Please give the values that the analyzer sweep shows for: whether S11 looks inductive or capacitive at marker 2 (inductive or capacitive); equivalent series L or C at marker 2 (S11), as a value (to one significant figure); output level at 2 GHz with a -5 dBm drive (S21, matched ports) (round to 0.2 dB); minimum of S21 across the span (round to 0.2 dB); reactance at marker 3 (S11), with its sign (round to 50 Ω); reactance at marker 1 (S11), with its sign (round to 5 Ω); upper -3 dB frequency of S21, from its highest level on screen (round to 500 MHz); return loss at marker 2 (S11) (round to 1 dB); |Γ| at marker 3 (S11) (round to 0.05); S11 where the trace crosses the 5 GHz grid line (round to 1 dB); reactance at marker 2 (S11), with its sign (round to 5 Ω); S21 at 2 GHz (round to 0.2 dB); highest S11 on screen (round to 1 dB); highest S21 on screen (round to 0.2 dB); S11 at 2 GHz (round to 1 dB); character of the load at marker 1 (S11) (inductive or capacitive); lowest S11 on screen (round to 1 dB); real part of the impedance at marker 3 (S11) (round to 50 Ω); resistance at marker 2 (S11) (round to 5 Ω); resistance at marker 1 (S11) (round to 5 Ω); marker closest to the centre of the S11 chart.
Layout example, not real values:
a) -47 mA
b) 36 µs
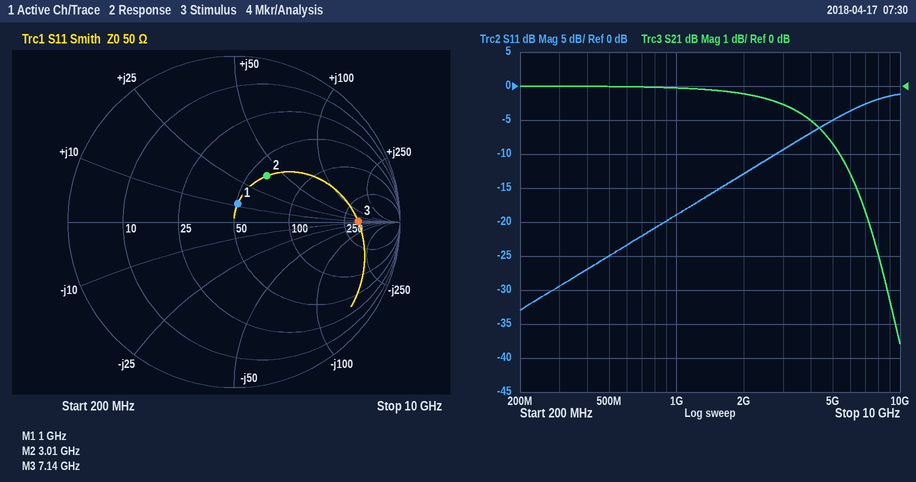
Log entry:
a) inductive
b) 2 nH
c) -5.2 dBm
d) -7.6 dB
e) 0 Ω
f) +10 Ω
g) 6.5 GHz
h) 9 dB
i) 0.75
j) -5 dB
k) +40 Ω
l) -0.2 dB
m) -1 dB
n) 0.0 dB
o) -13 dB
p) inductive
q) -33 dB
r) 350 Ω
s) 60 Ω
t) 50 Ω
u) marker 1
